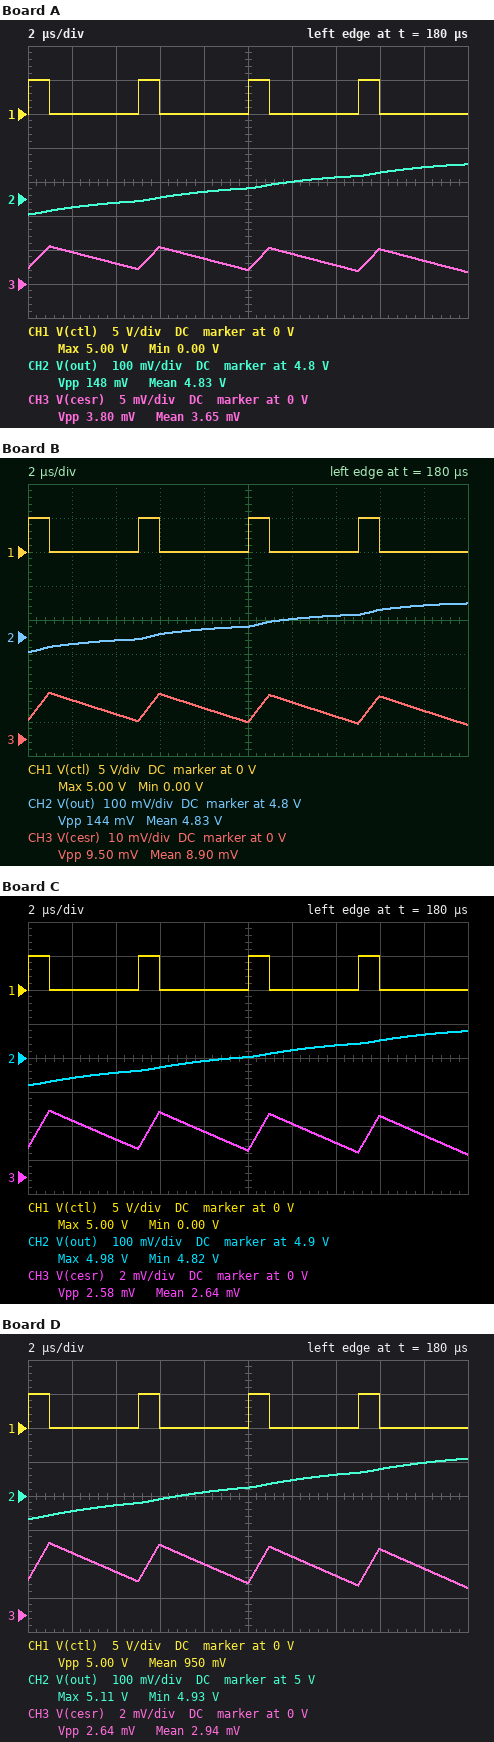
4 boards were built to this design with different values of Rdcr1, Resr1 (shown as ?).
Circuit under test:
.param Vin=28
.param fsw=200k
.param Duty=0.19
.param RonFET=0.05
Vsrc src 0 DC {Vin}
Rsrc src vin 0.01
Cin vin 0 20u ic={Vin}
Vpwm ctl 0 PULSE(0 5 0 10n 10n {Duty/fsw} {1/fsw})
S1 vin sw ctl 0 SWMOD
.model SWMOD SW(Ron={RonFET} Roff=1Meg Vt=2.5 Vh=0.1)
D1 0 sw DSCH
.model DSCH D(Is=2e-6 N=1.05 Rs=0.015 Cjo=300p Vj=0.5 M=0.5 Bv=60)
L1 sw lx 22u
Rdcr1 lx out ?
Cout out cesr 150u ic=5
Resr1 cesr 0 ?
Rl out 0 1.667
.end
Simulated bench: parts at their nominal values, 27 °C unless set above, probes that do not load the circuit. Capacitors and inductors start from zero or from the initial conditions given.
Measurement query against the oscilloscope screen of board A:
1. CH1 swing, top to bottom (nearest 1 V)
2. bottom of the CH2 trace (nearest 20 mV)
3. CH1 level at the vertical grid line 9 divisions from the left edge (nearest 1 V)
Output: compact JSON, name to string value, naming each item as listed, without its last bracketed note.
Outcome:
{"CH1 swing, top to bottom": "5 V", "bottom of the CH2 trace": "4.76 V", "CH1 level at the vertical grid line 9 divisions from the left edge": "0 V"}
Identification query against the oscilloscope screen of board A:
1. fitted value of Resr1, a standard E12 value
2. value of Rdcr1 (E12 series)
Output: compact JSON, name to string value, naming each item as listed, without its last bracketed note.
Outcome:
{"fitted value of Resr1, a standard E12 value": "3.3 mΩ", "value of Rdcr1": "0.056 Ω"}
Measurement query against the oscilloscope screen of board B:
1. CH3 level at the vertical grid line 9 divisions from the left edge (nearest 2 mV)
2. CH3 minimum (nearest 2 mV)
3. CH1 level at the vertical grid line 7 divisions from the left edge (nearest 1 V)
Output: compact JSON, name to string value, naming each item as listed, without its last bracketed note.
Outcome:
{"CH3 level at the vertical grid line 9 divisions from the left edge": "8 mV", "CH3 minimum": "4 mV", "CH1 level at the vertical grid line 7 divisions from the left edge": "0 V"}
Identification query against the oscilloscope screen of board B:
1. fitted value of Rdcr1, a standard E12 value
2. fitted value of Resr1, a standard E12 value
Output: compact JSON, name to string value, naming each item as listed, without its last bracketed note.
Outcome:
{"fitted value of Rdcr1, a standard E12 value": "0.056 Ω", "fitted value of Resr1, a standard E12 value": "8.2 mΩ"}
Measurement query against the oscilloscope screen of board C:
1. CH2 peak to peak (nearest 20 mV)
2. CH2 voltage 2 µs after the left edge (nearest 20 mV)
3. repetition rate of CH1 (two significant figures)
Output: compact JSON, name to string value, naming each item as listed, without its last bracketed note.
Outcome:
{"CH2 peak to peak": "160 mV", "CH2 voltage 2 µs after the left edge": "4.84 V", "repetition rate of CH1": "200 kHz"}
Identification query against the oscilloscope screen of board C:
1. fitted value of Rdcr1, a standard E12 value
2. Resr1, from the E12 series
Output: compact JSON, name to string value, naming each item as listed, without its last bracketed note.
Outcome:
{"fitted value of Rdcr1, a standard E12 value": "0.039 Ω", "Resr1, from the E12 series": "2.2 mΩ"}
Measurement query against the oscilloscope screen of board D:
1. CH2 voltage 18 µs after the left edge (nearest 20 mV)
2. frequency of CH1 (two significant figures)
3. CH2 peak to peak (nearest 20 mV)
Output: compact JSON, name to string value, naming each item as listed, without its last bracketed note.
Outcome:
{"CH2 voltage 18 µs after the left edge": "5.10 V", "frequency of CH1": "200 kHz", "CH2 peak to peak": "180 mV"}
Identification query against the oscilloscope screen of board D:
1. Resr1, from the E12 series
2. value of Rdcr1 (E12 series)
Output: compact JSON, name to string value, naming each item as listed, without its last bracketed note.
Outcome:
{"Resr1, from the E12 series": "2.2 mΩ", "value of Rdcr1": "0.012 Ω"}
